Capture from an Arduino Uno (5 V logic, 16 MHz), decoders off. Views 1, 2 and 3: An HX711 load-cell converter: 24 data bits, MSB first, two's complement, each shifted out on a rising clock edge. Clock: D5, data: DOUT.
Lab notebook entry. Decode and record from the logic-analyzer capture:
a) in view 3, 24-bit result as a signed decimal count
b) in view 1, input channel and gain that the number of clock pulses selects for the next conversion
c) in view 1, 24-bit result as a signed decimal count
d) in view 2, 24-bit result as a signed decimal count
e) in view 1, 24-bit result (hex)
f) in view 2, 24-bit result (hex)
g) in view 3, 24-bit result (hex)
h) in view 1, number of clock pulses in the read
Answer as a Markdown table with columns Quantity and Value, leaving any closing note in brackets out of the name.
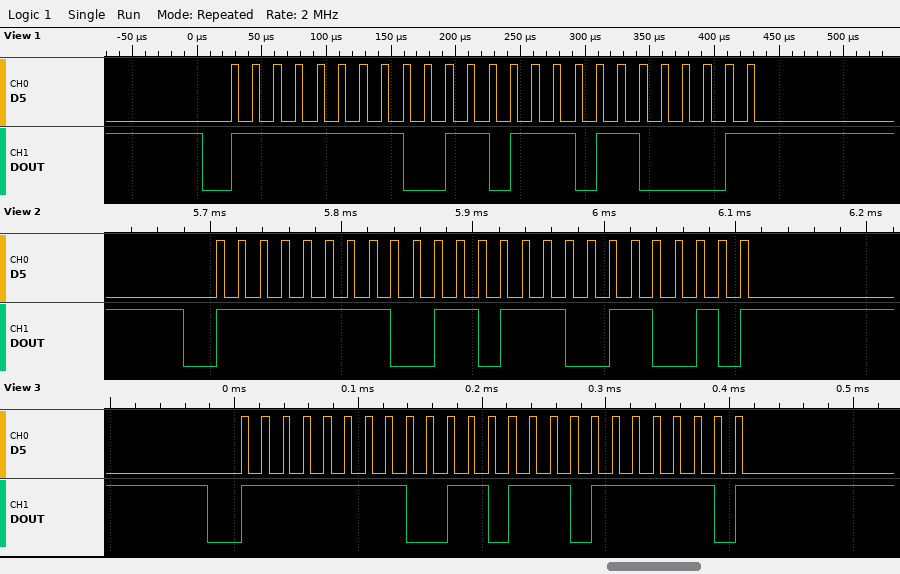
| Quantity | Value |
|---|---|
| in view 3, 24-bit result as a signed decimal count | -51330 |
| in view 1, input channel and gain that the number of clock pulses selects for the next conversion | channel A, gain 128 |
| in view 1, 24-bit result as a signed decimal count | -51359 |
| in view 2, 24-bit result as a signed decimal count | -51406 |
| in view 1, 24-bit result | 0xFF3761 |
| in view 2, 24-bit result | 0xFF3732 |
| in view 3, 24-bit result | 0xFF377E |
| in view 1, number of clock pulses in the read | 25 |
